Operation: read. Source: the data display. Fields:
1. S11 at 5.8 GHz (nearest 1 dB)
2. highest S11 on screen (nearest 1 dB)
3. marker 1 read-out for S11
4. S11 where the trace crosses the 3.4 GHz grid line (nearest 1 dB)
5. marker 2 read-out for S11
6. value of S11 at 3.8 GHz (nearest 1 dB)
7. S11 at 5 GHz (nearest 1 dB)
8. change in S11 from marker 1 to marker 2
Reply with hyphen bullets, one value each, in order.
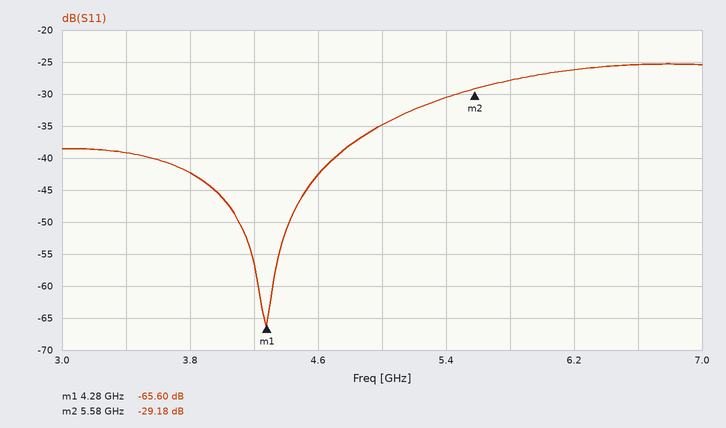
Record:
- -28 dB
- -25 dB
- -65.60 dB
- -39 dB
- -29.18 dB
- -42 dB
- -35 dB
- 36.42 dB
